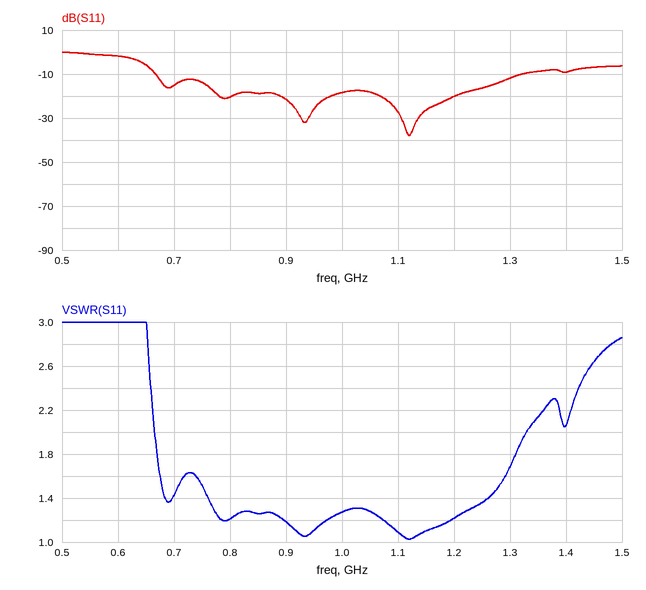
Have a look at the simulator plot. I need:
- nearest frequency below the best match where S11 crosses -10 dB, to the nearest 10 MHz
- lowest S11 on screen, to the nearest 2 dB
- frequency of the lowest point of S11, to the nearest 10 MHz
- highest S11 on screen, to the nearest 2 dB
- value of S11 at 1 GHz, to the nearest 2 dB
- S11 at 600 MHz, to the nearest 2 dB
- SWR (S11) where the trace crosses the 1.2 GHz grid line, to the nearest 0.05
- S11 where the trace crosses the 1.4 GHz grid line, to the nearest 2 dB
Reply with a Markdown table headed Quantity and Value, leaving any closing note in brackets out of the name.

| Quantity | Value |
|---|---|
| nearest frequency below the best match where S11 crosses -10 dB, to the nearest 10 MHz | 670 MHz |
| lowest S11 on screen, to the nearest 2 dB | -38 dB |
| frequency of the lowest point of S11, to the nearest 10 MHz | 1.12 GHz |
| highest S11 on screen, to the nearest 2 dB | 0 dB |
| value of S11 at 1 GHz, to the nearest 2 dB | -18 dB |
| S11 at 600 MHz, to the nearest 2 dB | -2 dB |
| SWR (S11) where the trace crosses the 1.2 GHz grid line, to the nearest 0.05 | 1.20 |
| S11 where the trace crosses the 1.4 GHz grid line, to the nearest 2 dB | -10 dB |
